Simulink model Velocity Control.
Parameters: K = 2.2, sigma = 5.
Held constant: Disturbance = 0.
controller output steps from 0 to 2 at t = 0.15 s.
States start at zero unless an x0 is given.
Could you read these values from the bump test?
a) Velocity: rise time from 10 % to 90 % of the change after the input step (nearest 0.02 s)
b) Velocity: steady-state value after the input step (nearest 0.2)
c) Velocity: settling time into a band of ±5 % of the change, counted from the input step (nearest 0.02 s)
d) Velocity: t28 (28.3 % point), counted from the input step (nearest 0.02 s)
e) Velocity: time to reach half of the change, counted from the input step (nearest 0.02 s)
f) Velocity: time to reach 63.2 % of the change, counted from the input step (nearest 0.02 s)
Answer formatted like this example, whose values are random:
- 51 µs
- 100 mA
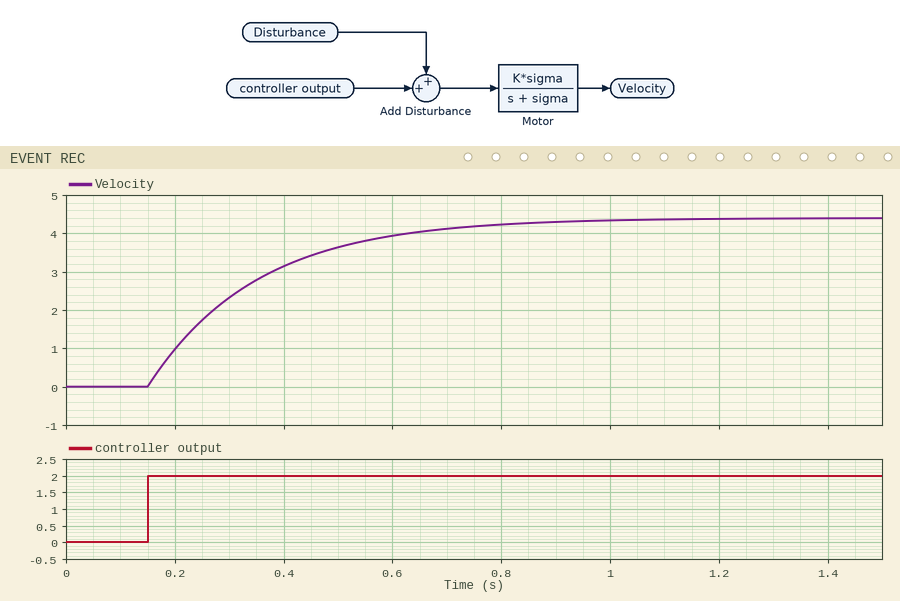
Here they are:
- 0.44 s
- 4.4
- 0.60 s
- 0.06 s
- 0.14 s
- 0.20 s
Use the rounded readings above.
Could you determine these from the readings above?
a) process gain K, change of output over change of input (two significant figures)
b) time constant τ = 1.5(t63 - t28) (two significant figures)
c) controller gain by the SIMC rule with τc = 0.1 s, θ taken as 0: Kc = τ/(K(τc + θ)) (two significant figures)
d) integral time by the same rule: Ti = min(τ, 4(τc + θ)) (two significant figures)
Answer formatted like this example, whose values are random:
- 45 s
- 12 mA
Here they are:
- 2.2
- 0.21 s
- 0.95
- 0.21 s
